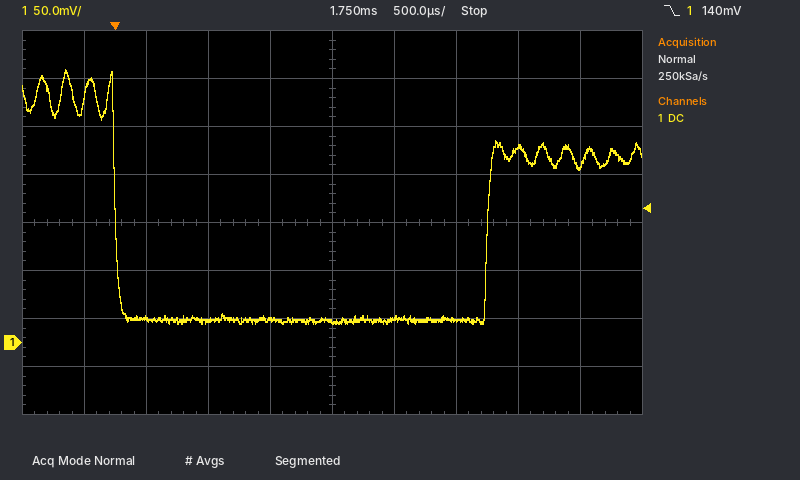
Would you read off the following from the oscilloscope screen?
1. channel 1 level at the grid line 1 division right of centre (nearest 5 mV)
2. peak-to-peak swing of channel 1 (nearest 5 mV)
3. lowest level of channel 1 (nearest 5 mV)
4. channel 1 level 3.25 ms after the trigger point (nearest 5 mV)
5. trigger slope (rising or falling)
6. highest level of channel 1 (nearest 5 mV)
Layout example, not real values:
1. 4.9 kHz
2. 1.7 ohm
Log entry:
1. 25 mV
2. 265 mV
3. 20 mV
4. 200 mV
5. falling
6. 285 mV
